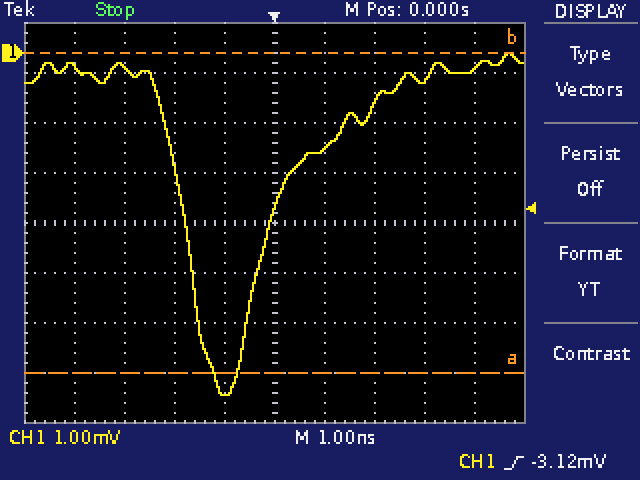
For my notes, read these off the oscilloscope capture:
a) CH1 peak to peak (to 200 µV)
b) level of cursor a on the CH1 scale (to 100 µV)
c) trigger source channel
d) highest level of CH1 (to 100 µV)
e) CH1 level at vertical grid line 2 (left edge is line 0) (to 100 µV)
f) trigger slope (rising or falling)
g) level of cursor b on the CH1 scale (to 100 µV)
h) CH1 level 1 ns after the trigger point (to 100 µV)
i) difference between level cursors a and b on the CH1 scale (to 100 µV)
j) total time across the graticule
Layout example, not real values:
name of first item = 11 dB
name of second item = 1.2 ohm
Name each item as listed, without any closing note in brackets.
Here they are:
CH1 peak to peak = 6.8 mV
level of cursor a on the CH1 scale = -6.4 mV
trigger source channel = CH1
highest level of CH1 = 0.0 mV
CH1 level at vertical grid line 2 (left edge is line 0) = -300 µV
trigger slope = rising
level of cursor b on the CH1 scale = 0.0 mV
CH1 level 1 ns after the trigger point = -1.9 mV
difference between level cursors a and b on the CH1 scale = 6.4 mV
total time across the graticule = 10 ns
